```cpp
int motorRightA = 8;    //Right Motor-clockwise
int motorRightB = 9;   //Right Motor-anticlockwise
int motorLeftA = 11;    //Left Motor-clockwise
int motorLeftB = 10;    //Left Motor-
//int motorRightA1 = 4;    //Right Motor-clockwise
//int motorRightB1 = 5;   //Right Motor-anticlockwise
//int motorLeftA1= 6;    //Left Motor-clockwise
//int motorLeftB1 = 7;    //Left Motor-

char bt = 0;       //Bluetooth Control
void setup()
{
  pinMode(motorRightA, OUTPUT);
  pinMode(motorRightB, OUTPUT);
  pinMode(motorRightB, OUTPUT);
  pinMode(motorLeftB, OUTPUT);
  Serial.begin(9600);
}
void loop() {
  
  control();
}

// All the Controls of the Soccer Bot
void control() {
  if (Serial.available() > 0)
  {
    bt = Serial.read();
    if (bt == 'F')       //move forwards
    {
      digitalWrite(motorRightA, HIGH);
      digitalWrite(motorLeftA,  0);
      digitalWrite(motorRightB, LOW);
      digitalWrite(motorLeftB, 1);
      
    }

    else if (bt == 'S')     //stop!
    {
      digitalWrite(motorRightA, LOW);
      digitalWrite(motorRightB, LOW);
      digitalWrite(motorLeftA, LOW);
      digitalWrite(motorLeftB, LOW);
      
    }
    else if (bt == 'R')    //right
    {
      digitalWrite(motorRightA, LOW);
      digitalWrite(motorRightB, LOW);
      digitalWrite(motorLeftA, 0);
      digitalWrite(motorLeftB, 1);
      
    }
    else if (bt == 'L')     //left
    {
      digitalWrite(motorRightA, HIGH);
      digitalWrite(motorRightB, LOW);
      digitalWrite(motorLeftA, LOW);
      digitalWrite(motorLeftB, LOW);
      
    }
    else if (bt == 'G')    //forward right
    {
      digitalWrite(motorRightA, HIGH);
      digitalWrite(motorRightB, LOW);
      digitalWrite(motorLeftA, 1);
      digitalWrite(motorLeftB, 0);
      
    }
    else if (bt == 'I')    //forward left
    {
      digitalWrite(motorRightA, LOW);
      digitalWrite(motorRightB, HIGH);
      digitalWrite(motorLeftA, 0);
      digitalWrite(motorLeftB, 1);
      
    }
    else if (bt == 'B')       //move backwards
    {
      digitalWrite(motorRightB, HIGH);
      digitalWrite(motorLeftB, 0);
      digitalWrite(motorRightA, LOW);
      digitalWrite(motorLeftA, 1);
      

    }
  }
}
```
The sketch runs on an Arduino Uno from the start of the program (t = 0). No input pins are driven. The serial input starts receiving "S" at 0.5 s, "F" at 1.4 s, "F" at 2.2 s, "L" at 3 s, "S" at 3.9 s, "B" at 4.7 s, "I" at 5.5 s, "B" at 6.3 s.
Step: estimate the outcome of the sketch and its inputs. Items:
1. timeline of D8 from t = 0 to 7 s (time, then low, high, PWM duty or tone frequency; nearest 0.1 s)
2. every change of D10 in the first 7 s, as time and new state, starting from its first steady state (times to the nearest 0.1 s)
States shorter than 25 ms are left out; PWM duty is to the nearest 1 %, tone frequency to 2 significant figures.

0 s low; 1.4 s high; 3.9 s low
0 s low; 1.4 s high; 3 s low; 5.5 s high; 6.3 s low
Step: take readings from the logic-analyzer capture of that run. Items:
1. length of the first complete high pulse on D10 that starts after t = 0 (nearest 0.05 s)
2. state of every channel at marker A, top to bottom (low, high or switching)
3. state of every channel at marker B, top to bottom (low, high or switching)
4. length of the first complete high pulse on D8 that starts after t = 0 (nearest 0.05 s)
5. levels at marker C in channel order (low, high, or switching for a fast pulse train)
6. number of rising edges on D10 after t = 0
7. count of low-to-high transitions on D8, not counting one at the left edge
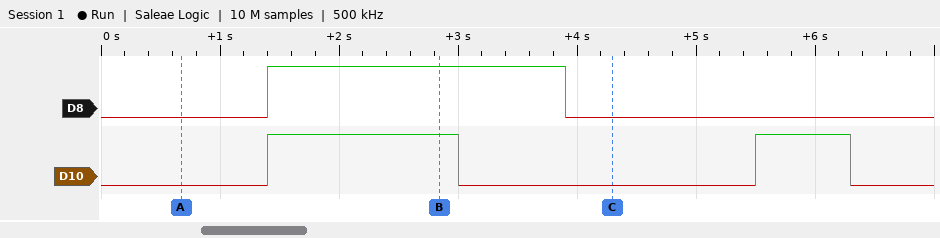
1.60 s
D8 low, D10 low
D8 high, D10 high
2.50 s
D8 low, D10 low
2
1
